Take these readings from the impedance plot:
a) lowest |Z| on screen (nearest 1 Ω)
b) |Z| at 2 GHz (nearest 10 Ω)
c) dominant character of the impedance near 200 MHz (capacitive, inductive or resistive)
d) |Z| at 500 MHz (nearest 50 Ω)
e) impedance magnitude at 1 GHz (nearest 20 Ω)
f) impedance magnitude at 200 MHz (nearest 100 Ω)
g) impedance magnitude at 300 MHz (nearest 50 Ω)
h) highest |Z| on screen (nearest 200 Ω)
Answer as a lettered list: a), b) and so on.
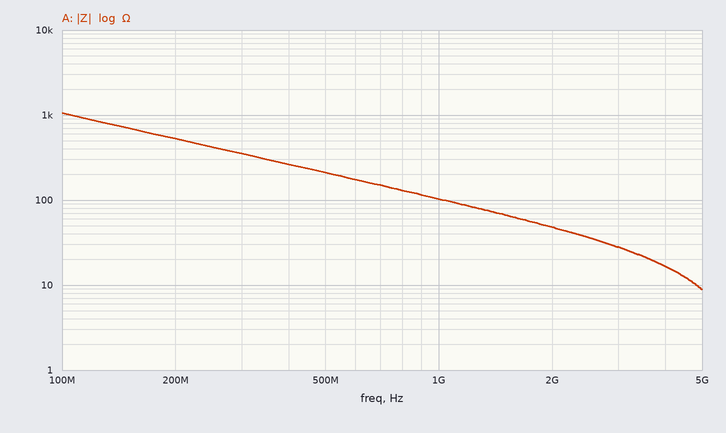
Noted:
a) 9 Ω
b) 50 Ω
c) capacitive
d) 200 Ω
e) 100 Ω
f) 500 Ω
g) 350 Ω
h) 1.0 kΩ
